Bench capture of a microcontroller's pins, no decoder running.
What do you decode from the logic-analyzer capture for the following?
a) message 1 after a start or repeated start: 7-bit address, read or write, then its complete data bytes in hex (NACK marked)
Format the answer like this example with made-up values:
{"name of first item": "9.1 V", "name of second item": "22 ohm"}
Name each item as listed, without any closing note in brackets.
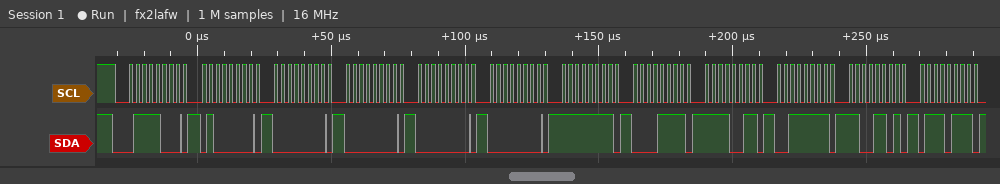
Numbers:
{"message 1 after a start or repeated start: 7-bit address, read or write, then its complete data bytes in hex": "0x3C write: 40 00 00 00 00 FF 0F F3 3F CD 77"}
